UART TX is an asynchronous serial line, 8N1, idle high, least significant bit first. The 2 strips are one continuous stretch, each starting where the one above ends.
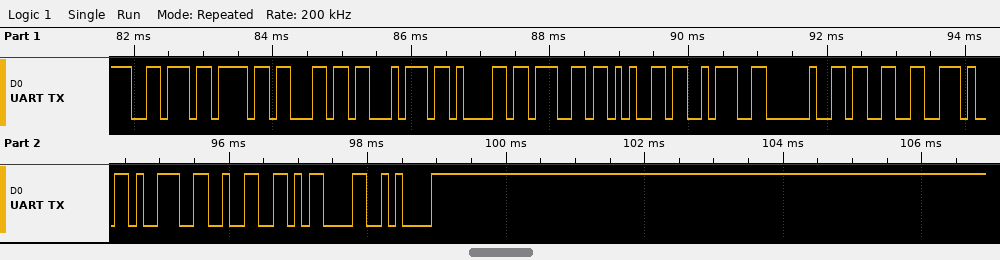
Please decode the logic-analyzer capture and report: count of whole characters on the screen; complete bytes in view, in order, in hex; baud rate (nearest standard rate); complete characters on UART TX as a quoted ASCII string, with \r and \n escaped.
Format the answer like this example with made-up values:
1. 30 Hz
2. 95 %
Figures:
1. 15
2. 0x76 0x6F 0x6C 0x74 0x61 0x67 0x65 0x3A 0x20 0x33 0x2E 0x39 0x32 0x0D 0x0A
3. 9600 baud
4. "voltage: 3.92\r\n"
